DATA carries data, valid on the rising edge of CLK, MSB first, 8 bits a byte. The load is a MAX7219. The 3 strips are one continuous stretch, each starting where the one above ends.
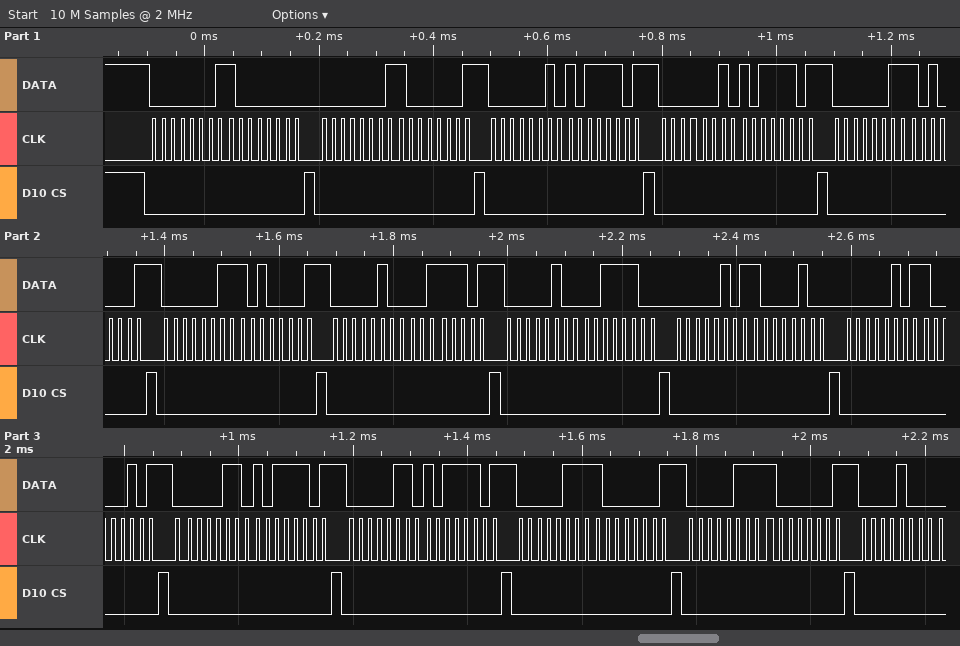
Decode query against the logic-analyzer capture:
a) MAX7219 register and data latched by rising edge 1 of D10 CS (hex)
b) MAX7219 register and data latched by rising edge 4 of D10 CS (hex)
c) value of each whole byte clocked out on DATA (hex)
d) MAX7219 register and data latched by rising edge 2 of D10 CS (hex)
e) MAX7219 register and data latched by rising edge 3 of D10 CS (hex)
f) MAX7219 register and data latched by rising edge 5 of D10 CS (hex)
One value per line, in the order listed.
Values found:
register 0x1, data 0x80
register 0x2, data 0xBD
0x01 0x80 0x01 0x81 0x02 0xBD 0x02 0xBD 0x03 0xA1 0x03 0xA1 0x04 0x3D 0x04 0x3C 0x05 0x84 0x05 0x85 0x06 0xBD 0x06 0xBD 0x07 0x81 0x07 0x81 0x08
register 0x1, data 0x81
register 0x2, data 0xBD
register 0x3, data 0xA1
